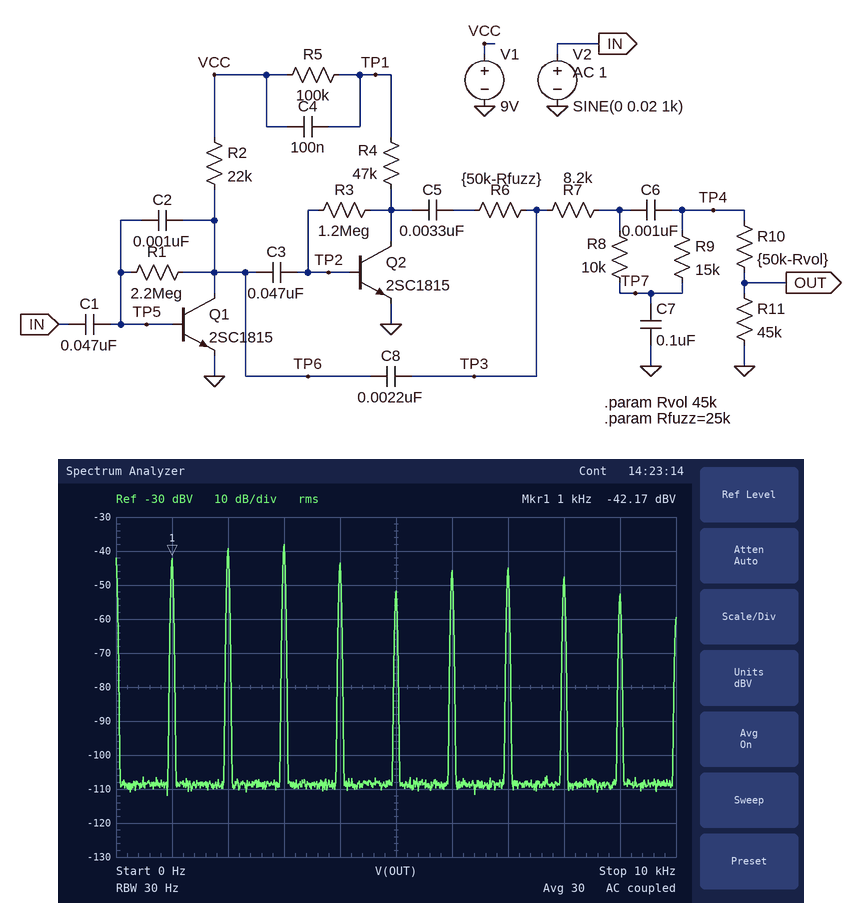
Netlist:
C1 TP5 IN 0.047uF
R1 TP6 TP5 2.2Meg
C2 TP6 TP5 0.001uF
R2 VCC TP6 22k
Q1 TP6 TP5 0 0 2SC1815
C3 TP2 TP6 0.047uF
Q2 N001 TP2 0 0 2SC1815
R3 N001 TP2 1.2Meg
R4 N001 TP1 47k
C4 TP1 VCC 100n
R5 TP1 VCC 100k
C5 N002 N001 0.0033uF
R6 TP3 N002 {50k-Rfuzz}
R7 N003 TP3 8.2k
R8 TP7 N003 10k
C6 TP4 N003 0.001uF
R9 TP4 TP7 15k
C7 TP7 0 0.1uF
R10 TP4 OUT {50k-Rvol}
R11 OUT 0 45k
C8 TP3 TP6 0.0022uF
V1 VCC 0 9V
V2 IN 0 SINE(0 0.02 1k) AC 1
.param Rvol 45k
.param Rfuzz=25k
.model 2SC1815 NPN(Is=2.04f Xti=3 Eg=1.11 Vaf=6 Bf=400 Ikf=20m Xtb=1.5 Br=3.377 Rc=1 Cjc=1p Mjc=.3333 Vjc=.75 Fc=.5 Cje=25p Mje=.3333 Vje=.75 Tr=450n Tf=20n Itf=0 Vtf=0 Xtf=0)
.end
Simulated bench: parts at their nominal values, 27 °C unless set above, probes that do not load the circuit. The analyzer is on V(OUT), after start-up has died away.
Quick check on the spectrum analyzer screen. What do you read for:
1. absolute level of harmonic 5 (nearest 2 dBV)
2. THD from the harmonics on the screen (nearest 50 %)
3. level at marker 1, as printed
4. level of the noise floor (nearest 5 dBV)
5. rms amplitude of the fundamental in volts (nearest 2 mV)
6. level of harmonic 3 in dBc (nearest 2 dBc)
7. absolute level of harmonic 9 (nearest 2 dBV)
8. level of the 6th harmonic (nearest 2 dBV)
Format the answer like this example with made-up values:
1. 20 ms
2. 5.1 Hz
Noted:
1. -52 dBV
2. 250 %
3. -42.17 dBV
4. -110 dBV
5. 8 mV
6. 4 dBc
7. -52 dBV
8. -46 dBV
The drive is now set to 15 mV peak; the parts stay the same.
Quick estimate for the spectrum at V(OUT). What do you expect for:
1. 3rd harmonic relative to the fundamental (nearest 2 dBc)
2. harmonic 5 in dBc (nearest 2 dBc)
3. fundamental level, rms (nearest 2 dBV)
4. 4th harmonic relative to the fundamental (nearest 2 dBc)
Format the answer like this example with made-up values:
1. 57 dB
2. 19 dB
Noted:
1. 2 dBc
2. -8 dBc
3. -42 dBV
4. -6 dBc
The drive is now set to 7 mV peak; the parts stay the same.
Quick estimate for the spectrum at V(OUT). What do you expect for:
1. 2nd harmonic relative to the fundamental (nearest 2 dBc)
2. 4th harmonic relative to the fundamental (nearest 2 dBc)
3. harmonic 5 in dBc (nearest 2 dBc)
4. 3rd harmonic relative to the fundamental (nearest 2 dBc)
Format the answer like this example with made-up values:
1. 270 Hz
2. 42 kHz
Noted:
1. 0 dBc
2. -10 dBc
3. -6 dBc
4. -4 dBc
